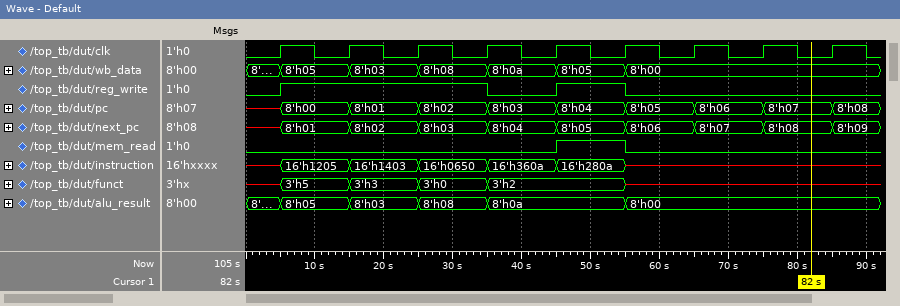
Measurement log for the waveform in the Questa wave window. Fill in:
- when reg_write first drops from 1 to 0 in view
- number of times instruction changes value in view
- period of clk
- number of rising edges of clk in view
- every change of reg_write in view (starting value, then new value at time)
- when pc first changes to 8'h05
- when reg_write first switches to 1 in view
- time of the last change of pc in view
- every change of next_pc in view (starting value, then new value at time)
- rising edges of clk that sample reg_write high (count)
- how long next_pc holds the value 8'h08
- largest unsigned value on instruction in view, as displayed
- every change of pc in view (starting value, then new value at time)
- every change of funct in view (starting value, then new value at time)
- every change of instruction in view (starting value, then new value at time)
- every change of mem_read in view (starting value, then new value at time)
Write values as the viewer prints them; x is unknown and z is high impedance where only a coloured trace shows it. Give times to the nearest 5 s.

35 s
6
10 s
9
0, 1 at 5 s, 0 at 35 s, 1 at 45 s, 0 at 55 s
55 s
5 s
85 s
x, 8'h01 at 5 s, 8'h02 at 15 s, 8'h03 at 25 s, 8'h04 at 35 s, 8'h05 at 45 s, 8'h06 at 55 s, 8'h07 at 65 s, 8'h08 at 75 s, 8'h09 at 85 s
4
10 s
16'h360a
x, 8'h00 at 5 s, 8'h01 at 15 s, 8'h02 at 25 s, 8'h03 at 35 s, 8'h04 at 45 s, 8'h05 at 55 s, 8'h06 at 65 s, 8'h07 at 75 s, 8'h08 at 85 s
x, 3'h5 at 5 s, 3'h3 at 15 s, 3'h0 at 25 s, 3'h2 at 35 s, x at 55 s
x, 16'h1205 at 5 s, 16'h1403 at 15 s, 16'h0650 at 25 s, 16'h360a at 35 s, 16'h280a at 45 s, x at 55 s
0, 1 at 45 s, 0 at 55 s
